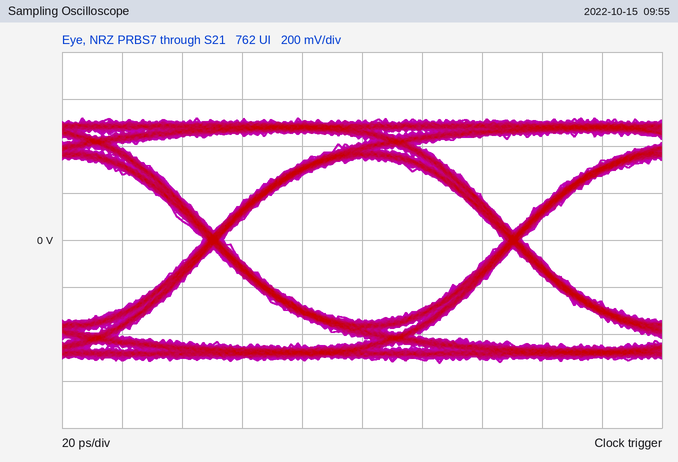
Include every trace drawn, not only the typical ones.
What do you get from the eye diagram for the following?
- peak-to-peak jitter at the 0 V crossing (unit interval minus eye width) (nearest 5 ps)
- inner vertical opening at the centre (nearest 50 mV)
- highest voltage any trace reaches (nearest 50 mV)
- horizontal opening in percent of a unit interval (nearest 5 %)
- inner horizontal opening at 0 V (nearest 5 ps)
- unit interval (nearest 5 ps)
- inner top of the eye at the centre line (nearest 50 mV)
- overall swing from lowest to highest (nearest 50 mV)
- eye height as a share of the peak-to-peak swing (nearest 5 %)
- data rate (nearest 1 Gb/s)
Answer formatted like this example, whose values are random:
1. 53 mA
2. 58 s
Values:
1. 5 ps
2. 700 mV
3. 500 mV
4. 95 %
5. 95 ps
6. 100 ps
7. 350 mV
8. 1.05 V
9. 65 %
10. 10 Gb/s
